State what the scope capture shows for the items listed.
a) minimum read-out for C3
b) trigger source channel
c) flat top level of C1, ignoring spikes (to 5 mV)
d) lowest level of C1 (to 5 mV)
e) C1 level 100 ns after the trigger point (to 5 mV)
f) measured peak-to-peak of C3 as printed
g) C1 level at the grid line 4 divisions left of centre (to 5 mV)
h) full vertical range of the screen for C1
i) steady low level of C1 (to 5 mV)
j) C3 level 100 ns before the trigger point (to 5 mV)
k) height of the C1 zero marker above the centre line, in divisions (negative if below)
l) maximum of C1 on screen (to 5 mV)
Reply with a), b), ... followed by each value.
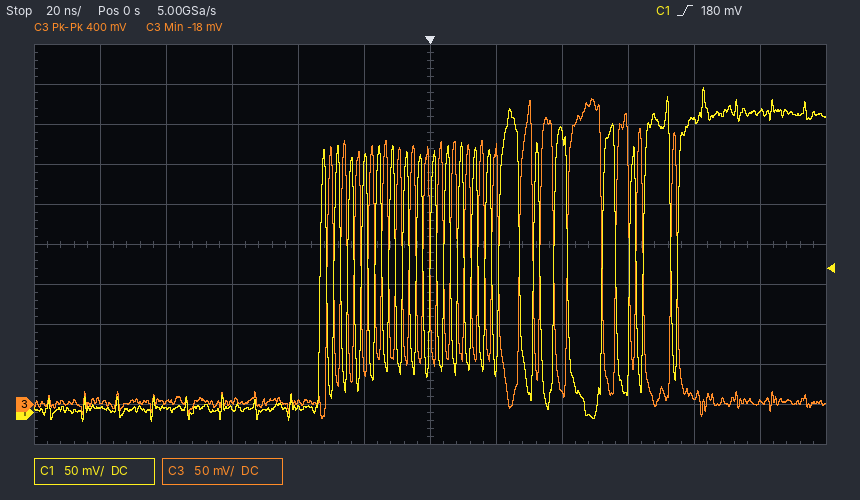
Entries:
a) -18 mV
b) C1
c) 375 mV
d) -10 mV
e) 375 mV
f) 400 mV
g) 5 mV
h) 500 mV
i) 5 mV
j) 5 mV
k) -4.2 div
l) 405 mV
